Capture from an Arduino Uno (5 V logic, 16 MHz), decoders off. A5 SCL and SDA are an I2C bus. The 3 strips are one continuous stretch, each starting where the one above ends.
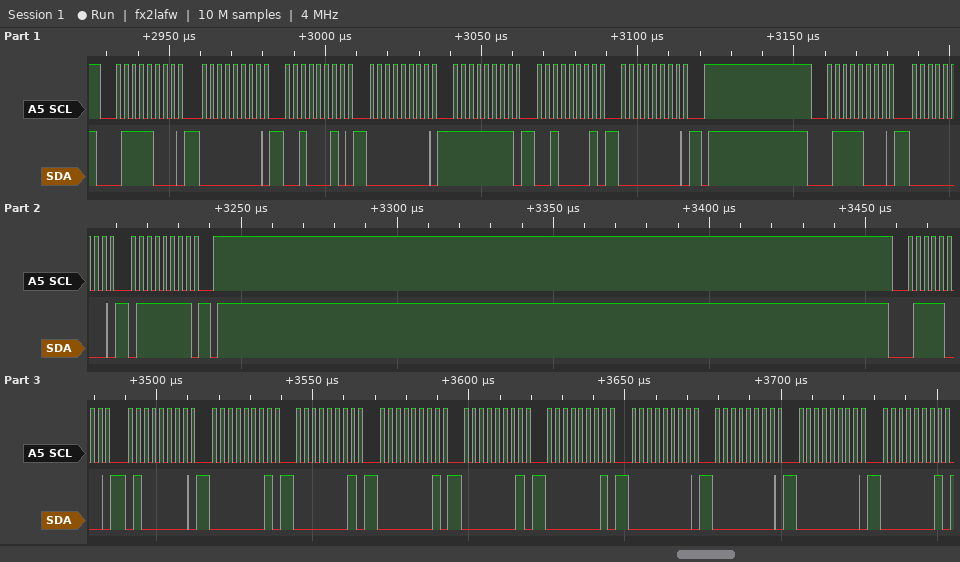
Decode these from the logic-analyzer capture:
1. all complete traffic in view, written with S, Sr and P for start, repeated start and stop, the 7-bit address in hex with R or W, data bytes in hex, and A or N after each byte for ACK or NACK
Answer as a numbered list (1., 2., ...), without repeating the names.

1. S 3CW A 00 A 22 A 00 A FF A 21 A 00 A P S 3CW A 00 A 7F A P S 3CW A 40 A 01 A 01 A 01 A 01 A 01 A 00 A 00 A 00 A 01 A
